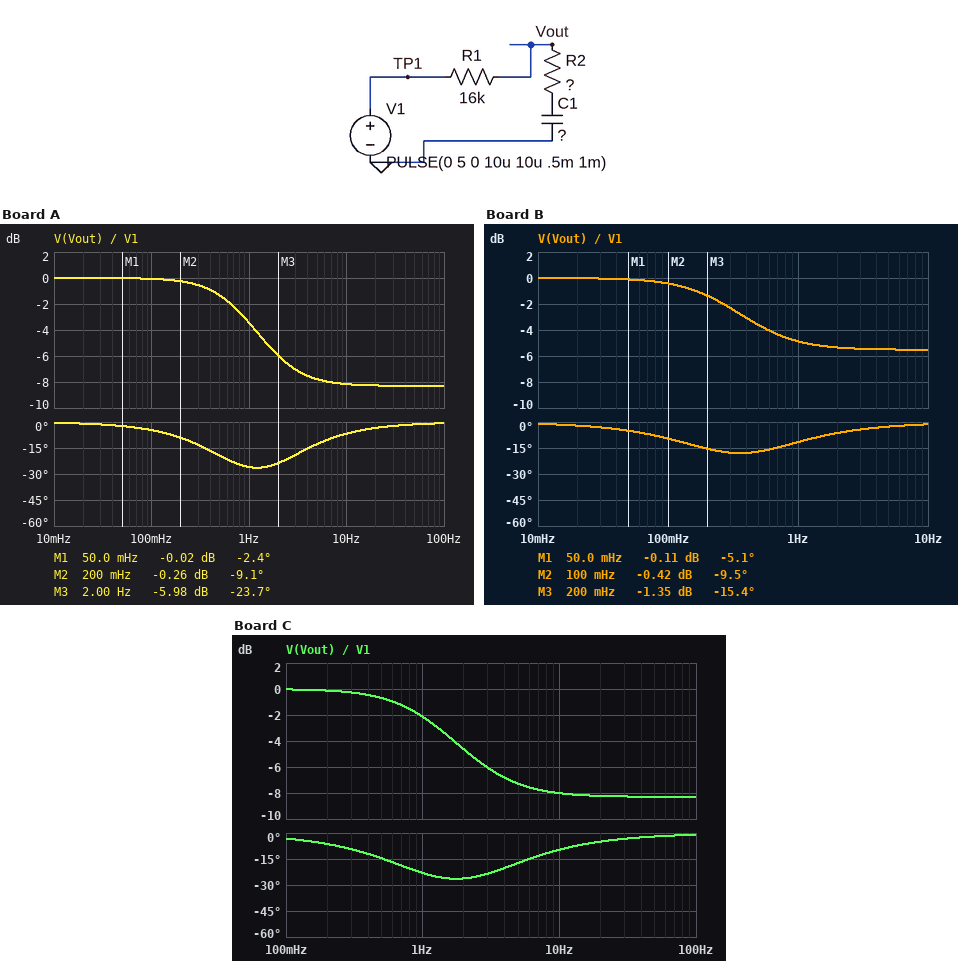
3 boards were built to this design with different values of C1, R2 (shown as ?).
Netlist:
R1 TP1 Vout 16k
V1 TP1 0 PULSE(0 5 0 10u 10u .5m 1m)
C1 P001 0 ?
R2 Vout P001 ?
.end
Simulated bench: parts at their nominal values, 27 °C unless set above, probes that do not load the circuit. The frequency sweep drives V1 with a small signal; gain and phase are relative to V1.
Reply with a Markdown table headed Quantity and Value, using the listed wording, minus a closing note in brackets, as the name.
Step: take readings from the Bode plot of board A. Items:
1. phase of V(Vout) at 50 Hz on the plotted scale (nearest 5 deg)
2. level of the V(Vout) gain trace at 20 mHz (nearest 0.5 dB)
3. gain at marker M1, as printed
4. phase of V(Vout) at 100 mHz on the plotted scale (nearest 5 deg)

| Quantity | Value |
|---|---|
| phase of V(Vout) at 50 Hz on the plotted scale | 0 deg |
| level of the V(Vout) gain trace at 20 mHz | 0 dB |
| gain at marker M1, as printed | -0.02 dB |
| phase of V(Vout) at 100 mHz on the plotted scale | -5 deg |
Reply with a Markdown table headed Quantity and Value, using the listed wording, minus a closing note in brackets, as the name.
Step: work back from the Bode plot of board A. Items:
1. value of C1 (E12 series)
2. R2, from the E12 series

| Quantity | Value |
|---|---|
| value of C1 | 8.2 µF |
| R2, from the E12 series | 10 kΩ |
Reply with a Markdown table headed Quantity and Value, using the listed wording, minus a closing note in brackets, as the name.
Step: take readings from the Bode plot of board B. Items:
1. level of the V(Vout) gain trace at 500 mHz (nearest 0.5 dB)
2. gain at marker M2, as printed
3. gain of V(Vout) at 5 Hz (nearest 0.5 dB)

| Quantity | Value |
|---|---|
| level of the V(Vout) gain trace at 500 mHz | -3.5 dB |
| gain at marker M2, as printed | -0.42 dB |
| gain of V(Vout) at 5 Hz | -5.5 dB |
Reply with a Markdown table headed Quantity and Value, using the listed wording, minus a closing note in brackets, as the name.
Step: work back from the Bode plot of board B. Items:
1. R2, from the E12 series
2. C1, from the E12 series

| Quantity | Value |
|---|---|
| R2, from the E12 series | 18 kΩ |
| C1, from the E12 series | 18 µF |
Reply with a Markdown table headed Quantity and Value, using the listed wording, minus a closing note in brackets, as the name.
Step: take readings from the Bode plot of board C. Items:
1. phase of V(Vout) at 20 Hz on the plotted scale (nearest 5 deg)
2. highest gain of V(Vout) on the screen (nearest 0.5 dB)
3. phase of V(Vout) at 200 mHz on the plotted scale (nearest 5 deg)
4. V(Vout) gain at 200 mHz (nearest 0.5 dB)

| Quantity | Value |
|---|---|
| phase of V(Vout) at 20 Hz on the plotted scale | -5 deg |
| highest gain of V(Vout) on the screen | 0 dB |
| phase of V(Vout) at 200 mHz on the plotted scale | -5 deg |
| V(Vout) gain at 200 mHz | 0 dB |
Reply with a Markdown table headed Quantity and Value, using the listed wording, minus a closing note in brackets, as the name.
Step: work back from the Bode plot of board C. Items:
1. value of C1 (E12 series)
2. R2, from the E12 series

| Quantity | Value |
|---|---|
| value of C1 | 5.6 µF |
| R2, from the E12 series | 10 kΩ |
